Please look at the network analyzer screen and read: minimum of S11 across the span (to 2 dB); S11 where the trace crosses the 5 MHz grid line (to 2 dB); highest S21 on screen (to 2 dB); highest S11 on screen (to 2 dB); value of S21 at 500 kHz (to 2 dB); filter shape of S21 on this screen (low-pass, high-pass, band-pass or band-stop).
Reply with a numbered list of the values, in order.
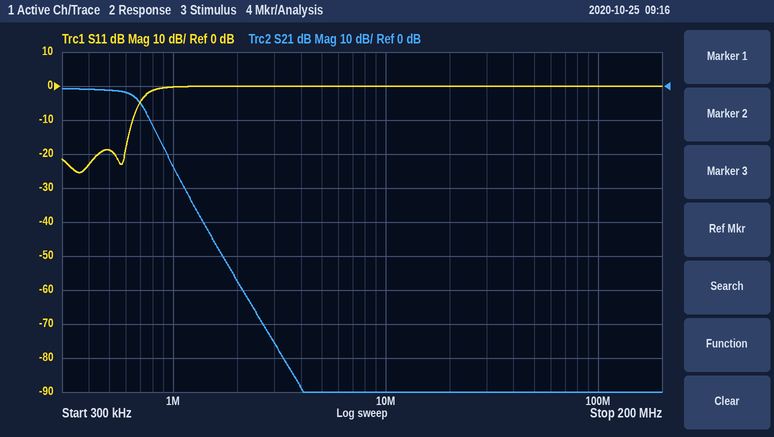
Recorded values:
1. -26 dB
2. 0 dB
3. 0 dB
4. 0 dB
5. -2 dB
6. low-pass
